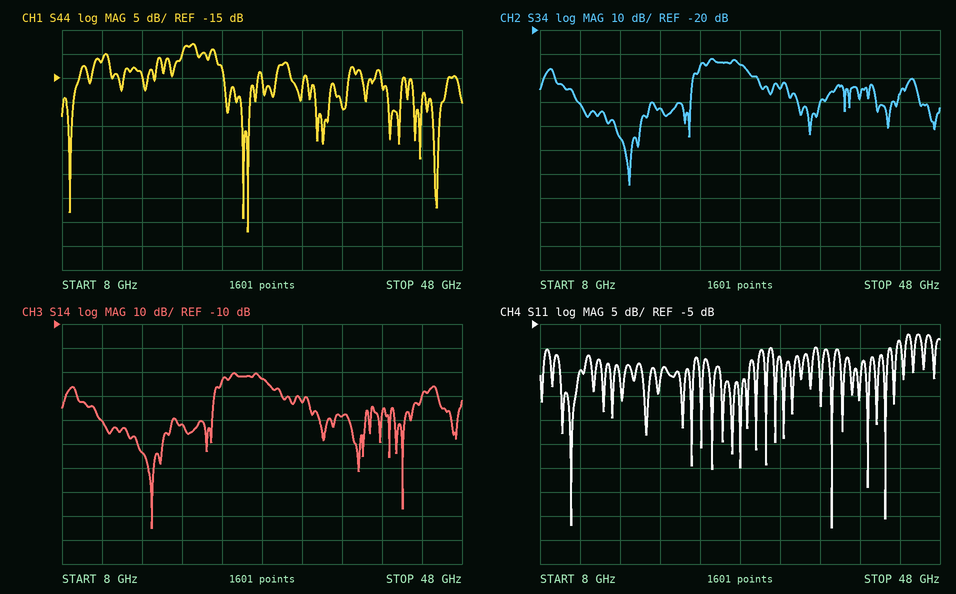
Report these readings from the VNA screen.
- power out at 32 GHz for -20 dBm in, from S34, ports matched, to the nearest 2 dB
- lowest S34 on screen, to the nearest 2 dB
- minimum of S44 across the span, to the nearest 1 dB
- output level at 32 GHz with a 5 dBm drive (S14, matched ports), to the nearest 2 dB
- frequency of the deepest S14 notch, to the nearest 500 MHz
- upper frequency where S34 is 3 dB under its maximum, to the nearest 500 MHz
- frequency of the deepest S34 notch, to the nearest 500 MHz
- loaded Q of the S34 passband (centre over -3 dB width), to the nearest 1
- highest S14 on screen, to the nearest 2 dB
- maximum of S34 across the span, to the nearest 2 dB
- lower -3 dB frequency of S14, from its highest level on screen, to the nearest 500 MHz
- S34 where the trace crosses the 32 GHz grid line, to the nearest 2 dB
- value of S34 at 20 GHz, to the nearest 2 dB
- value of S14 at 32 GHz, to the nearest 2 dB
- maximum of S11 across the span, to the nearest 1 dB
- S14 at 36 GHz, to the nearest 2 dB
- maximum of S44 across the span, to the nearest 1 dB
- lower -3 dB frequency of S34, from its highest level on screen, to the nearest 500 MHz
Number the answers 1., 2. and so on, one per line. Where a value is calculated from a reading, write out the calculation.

1. -20 dBm + (-44 dB) = -64 dBm
2. -84 dB
3. -47 dB
4. 5 dBm + (-42 dB) = -38 dBm
5. 17.0 GHz
6. 28.5 GHz
7. 17.0 GHz
8. 26.25 GHz / 4.5 GHz ≈ 6
9. -30 dB
10. -32 dB
11. 24.0 GHz
12. -44 dB
13. -52 dB
14. -42 dB
15. -7 dB
16. -48 dB
17. -8 dB
18. 24.0 GHz
